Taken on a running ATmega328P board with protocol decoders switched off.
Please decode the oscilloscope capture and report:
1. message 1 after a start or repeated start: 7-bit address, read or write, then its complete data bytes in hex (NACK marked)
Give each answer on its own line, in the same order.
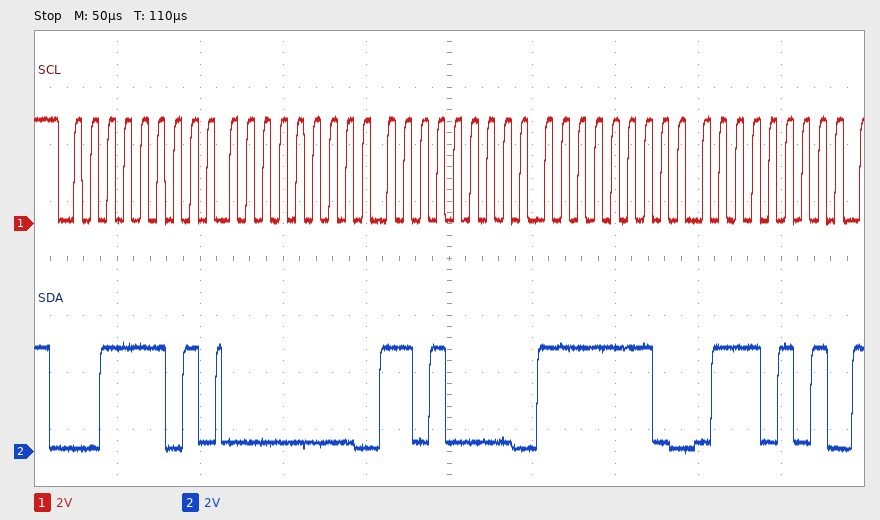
0x1E read: 00 D0 FE 75
